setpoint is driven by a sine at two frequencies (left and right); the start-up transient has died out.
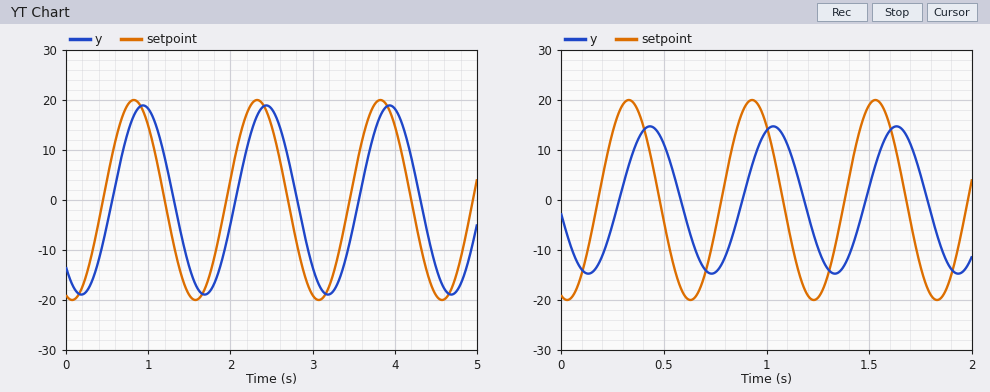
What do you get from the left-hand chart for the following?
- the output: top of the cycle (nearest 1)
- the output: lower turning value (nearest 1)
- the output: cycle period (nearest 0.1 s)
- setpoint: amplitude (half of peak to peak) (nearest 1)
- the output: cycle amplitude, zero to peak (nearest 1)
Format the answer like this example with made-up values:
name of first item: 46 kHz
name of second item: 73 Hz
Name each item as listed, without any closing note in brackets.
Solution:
the output: top of the cycle: 19
the output: lower turning value: -19
the output: cycle period: 1.5 s
setpoint: amplitude (half of peak to peak): 20
the output: cycle amplitude, zero to peak: 19
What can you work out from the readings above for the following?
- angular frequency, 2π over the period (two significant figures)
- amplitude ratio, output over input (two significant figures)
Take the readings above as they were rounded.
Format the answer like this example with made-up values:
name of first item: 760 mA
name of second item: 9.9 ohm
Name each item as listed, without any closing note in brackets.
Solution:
angular frequency, 2π over the period: 4.2 rad/s
amplitude ratio, output over input: 0.95
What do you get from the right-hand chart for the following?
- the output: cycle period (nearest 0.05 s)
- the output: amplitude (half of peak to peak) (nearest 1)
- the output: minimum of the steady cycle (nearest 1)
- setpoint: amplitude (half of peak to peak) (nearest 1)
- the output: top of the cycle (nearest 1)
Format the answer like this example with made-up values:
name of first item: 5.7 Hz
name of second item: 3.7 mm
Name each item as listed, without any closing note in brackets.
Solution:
the output: cycle period: 0.60 s
the output: amplitude (half of peak to peak): 15
the output: minimum of the steady cycle: -15
setpoint: amplitude (half of peak to peak): 20
the output: top of the cycle: 15
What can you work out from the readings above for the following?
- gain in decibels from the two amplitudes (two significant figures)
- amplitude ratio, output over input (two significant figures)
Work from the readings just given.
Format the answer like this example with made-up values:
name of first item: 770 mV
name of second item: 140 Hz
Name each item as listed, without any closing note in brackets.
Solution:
gain in decibels from the two amplitudes: -2.5 dB
amplitude ratio, output over input: 0.75
